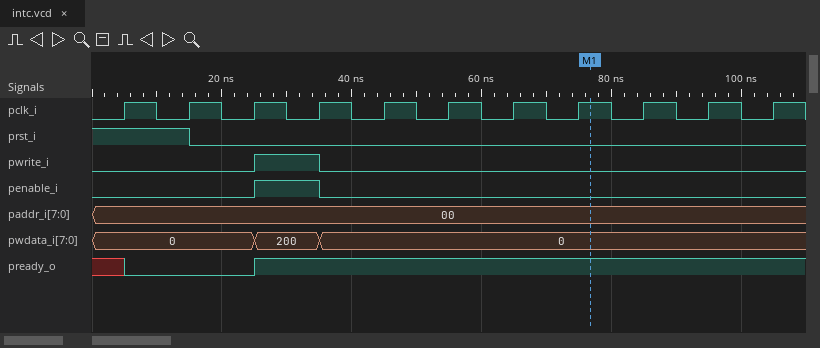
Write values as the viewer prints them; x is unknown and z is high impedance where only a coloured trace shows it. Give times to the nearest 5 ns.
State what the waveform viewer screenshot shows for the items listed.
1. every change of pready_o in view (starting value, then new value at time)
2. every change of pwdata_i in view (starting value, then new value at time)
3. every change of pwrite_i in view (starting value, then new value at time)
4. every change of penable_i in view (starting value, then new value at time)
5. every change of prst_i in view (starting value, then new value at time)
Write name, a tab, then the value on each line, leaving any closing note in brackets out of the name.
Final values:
every change of pready_o in view	x, 0 at 5 ns, 1 at 25 ns
every change of pwdata_i in view	0, 200 at 25 ns, 0 at 35 ns
every change of pwrite_i in view	0, 1 at 25 ns, 0 at 35 ns
every change of penable_i in view	0, 1 at 25 ns, 0 at 35 ns
every change of prst_i in view	1, 0 at 15 ns
